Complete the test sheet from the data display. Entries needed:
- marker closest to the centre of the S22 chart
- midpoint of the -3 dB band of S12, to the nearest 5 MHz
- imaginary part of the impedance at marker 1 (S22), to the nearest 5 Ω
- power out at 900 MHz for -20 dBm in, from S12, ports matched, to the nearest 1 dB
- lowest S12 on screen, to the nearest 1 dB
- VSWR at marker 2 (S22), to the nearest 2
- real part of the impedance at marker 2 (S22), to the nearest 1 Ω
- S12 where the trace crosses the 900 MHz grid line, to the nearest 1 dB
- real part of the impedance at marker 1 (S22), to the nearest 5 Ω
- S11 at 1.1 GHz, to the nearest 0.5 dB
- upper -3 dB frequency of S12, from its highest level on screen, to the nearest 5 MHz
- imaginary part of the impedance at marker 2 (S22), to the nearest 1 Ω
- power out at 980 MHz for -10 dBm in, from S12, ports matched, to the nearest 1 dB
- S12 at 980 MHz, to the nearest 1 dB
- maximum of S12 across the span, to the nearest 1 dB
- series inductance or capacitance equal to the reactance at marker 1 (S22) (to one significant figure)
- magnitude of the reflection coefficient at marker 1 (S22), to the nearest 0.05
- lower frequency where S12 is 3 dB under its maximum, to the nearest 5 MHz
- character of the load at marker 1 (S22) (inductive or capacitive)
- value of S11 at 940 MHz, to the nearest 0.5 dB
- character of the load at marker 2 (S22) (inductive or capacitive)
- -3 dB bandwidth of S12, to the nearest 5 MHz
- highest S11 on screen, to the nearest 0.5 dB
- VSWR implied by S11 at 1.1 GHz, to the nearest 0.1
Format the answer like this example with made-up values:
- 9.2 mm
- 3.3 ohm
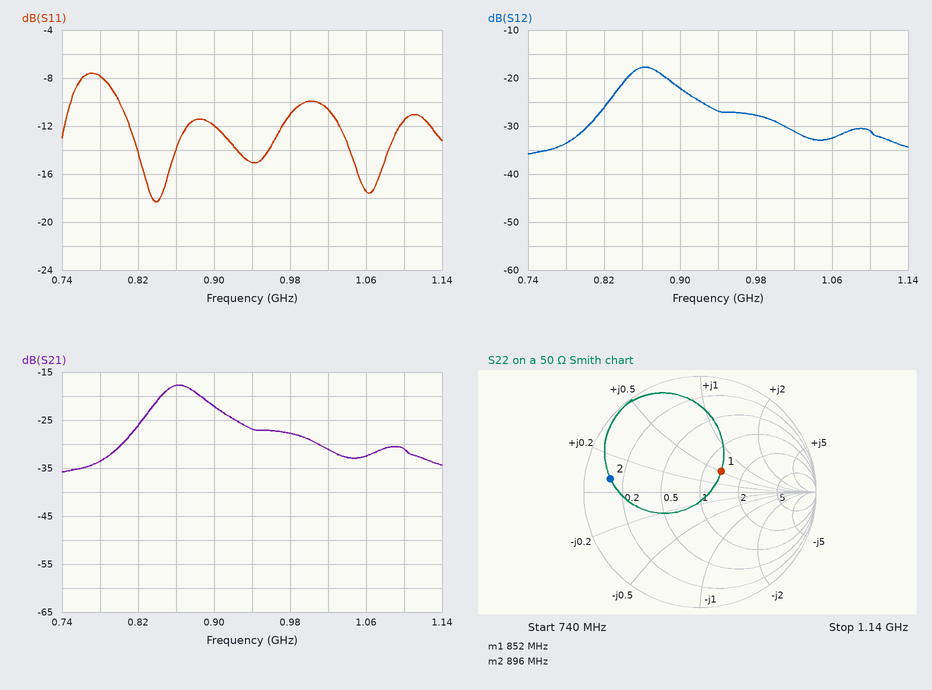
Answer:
- marker 1
- 865 MHz
- +25 Ω
- -42 dBm
- -36 dB
- 8
- 6 Ω
- -22 dB
- 65 Ω
- -11.5 dB
- 890 MHz
- +4 Ω
- -38 dBm
- -28 dB
- -18 dB
- 5 nH
- 0.25
- 840 MHz
- inductive
- -15.0 dB
- inductive
- 50 MHz
- -7.5 dB
- 1.7
